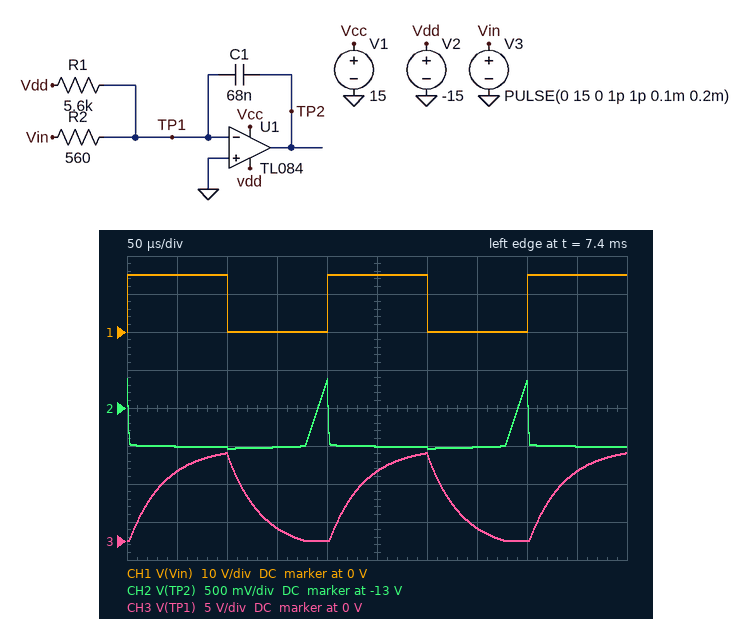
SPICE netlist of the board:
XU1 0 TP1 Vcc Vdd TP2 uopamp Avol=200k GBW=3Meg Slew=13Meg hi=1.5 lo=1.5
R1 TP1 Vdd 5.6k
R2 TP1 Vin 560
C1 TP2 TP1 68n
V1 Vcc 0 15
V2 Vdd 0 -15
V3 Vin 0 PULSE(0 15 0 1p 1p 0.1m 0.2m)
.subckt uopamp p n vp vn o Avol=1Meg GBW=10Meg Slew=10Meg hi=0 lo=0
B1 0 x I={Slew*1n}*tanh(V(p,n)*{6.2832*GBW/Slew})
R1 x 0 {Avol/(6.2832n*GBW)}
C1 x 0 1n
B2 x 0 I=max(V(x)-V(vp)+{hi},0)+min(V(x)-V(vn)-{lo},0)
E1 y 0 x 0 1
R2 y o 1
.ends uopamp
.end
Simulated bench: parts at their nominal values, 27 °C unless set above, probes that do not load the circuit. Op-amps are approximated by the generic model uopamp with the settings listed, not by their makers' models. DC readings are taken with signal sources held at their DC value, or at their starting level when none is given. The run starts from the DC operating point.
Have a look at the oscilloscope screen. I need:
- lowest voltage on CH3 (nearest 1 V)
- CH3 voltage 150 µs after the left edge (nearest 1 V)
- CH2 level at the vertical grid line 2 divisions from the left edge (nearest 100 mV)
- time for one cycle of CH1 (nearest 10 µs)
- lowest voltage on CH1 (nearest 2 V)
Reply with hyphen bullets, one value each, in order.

- 0 V
- 2 V
- -13.5 V
- 200 µs
- 0 V
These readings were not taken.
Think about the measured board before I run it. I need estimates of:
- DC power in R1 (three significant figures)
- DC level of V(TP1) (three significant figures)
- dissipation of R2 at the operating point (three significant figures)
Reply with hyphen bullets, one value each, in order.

- 33.2 mW
- -1.36 V
- 3.32 mW
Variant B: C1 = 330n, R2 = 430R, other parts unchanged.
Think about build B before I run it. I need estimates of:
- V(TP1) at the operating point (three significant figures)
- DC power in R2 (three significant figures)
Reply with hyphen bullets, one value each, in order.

- -1.07 V
- 2.66 mW
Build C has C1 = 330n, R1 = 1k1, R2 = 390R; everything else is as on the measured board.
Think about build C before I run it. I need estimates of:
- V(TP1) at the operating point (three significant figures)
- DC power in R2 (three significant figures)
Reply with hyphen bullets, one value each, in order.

- -3.93 V
- 39.5 mW
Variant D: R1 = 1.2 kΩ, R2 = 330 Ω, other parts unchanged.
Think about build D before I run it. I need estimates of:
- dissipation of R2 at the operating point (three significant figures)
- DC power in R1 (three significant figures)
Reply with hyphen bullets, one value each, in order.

- 31.7 mW
- 115 mW
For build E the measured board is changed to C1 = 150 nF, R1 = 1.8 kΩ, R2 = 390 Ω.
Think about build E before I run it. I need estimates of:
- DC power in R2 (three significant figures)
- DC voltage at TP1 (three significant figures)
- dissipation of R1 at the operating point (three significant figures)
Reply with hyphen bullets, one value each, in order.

- 18.3 mW
- -2.67 V
- 84.4 mW
